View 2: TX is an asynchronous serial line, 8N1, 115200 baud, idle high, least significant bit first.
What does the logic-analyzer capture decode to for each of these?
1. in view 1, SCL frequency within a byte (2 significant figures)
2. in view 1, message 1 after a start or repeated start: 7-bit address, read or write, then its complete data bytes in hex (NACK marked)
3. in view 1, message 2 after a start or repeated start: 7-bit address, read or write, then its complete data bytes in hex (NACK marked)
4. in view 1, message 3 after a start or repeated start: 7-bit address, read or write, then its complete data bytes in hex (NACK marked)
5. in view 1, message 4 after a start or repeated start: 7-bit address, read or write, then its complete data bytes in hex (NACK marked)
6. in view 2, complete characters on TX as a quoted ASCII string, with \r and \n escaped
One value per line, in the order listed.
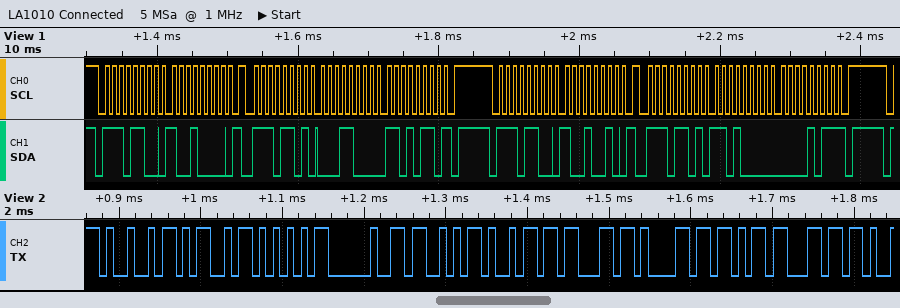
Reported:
100 kHz
0x76 write: 90
0x76 read: 18 D6 NACK
0x76 write: 92
0x76 read: D0 0B NACK
"IMU Sicakl"
